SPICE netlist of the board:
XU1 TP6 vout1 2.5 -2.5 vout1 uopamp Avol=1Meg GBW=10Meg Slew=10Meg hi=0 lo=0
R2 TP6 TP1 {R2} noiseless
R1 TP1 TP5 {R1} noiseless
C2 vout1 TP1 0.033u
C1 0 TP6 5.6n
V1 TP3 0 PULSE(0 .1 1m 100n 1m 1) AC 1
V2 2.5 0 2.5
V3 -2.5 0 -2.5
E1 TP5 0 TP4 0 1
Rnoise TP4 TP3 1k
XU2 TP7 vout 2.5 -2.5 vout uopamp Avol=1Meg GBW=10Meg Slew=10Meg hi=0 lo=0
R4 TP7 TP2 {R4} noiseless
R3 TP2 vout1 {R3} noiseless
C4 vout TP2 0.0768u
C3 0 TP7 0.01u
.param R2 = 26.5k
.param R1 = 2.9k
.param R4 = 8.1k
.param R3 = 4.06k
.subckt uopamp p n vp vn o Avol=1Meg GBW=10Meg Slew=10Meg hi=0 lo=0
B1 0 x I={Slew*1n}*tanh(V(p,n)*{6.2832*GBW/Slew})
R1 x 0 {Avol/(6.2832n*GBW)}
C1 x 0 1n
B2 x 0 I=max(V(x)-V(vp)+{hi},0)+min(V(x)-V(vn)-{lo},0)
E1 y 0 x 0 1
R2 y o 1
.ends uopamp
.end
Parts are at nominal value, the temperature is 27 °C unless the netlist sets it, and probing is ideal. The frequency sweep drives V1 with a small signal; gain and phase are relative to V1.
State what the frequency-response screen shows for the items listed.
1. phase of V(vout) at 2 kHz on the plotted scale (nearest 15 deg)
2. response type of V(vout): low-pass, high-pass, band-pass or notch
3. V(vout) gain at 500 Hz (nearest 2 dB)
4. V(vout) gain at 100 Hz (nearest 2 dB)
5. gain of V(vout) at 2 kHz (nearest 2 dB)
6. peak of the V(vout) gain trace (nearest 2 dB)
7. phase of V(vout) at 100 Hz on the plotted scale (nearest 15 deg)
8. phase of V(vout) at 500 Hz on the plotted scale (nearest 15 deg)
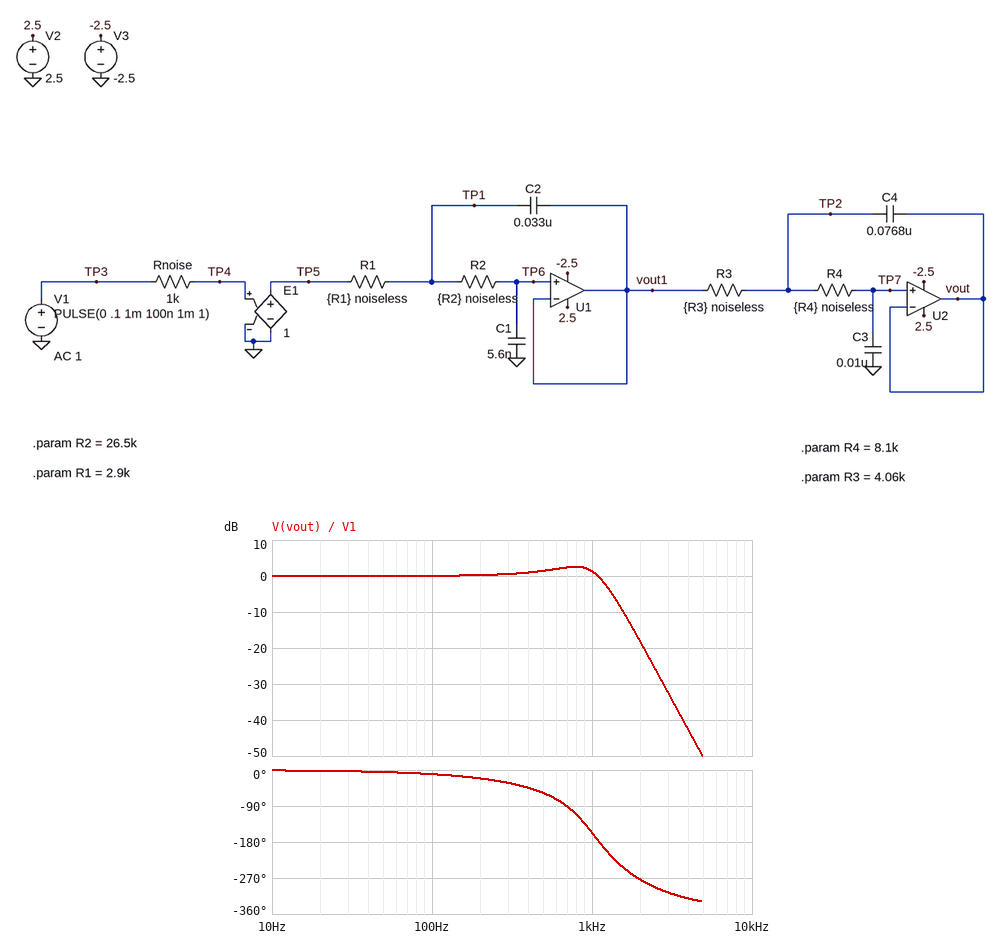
-270 deg
low-pass
2 dB
0 dB
-18 dB
2 dB
-15 deg
-60 deg
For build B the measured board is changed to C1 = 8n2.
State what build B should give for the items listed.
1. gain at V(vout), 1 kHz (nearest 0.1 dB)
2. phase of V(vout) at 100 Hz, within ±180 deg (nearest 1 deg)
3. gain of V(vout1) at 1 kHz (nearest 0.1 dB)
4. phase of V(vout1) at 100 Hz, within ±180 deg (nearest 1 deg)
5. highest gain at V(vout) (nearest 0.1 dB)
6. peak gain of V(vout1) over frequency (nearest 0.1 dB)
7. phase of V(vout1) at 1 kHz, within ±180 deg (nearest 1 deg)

-1.3 dB
-13 deg
-3.7 dB
-9 deg
0.9 dB
0 dB
-83 deg
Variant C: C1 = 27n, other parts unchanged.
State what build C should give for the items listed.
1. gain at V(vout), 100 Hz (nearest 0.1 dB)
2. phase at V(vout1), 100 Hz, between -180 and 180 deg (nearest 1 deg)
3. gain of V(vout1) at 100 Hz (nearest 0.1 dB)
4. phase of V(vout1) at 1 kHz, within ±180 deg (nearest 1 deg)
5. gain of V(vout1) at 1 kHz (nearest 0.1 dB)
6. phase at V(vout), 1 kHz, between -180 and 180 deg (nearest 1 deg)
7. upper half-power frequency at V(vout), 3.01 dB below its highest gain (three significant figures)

-0.7 dB
-27 deg
-0.8 dB
-109 deg
-14.4 dB
161 deg
243 Hz
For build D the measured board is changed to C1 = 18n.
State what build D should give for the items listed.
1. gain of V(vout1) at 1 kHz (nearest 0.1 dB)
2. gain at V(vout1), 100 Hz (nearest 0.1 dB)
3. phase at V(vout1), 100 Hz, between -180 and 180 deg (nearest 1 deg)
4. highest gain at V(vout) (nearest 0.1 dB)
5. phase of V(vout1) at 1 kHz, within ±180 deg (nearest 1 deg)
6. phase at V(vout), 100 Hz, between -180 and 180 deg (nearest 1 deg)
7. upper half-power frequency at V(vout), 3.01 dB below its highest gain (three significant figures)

-10.7 dB
-0.3 dB
-19 deg
0 dB
-104 deg
-23 deg
451 Hz
